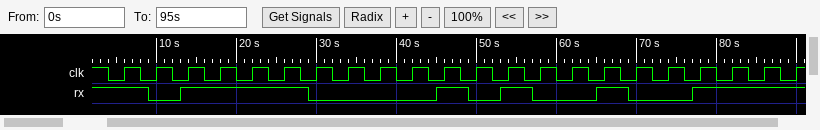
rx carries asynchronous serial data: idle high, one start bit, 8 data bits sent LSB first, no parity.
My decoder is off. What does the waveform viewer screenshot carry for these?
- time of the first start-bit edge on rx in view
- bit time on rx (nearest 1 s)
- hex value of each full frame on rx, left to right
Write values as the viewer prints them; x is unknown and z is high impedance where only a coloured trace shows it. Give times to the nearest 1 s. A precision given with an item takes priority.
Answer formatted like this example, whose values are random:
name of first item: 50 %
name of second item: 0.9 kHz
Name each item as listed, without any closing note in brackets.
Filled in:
time of the first start-bit edge on rx in view: 9 s
bit time on rx: 4 s
hex value of each full frame on rx, left to right: 0F, C9
